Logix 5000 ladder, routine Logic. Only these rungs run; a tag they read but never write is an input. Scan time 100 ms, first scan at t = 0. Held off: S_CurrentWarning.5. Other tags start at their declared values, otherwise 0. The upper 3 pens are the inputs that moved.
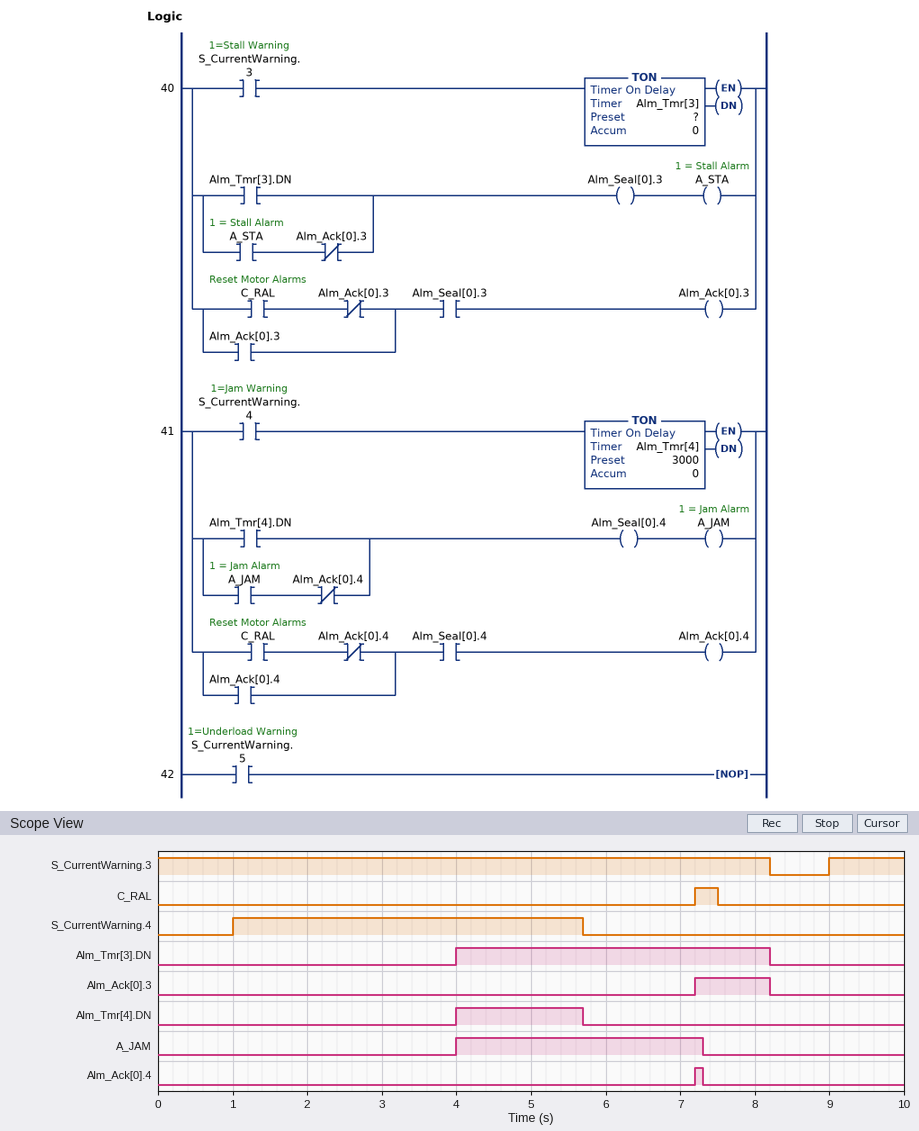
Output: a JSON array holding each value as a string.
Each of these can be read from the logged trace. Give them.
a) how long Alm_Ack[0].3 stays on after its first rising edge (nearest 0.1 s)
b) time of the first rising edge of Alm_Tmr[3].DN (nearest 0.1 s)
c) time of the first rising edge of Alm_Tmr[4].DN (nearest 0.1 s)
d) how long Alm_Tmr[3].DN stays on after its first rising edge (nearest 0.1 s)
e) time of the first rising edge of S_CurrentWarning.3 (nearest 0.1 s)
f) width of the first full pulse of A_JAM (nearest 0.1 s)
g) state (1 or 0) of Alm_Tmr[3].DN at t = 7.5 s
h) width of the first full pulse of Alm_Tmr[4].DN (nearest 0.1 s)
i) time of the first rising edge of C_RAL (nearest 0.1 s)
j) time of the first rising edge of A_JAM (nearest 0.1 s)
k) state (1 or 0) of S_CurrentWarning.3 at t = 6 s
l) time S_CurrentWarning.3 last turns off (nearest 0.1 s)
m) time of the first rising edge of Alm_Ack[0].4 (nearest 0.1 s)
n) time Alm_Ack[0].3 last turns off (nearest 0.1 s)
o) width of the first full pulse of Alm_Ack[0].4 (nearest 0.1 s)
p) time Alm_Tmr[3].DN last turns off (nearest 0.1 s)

["1.0 s", "4.0 s", "4.0 s", "4.2 s", "9.0 s", "3.3 s", "1", "1.7 s", "7.2 s", "4.0 s", "1", "8.2 s", "7.2 s", "8.2 s", "0.1 s", "8.2 s"]
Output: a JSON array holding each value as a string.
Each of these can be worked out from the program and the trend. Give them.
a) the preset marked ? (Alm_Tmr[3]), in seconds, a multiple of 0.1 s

["4.0 s"]
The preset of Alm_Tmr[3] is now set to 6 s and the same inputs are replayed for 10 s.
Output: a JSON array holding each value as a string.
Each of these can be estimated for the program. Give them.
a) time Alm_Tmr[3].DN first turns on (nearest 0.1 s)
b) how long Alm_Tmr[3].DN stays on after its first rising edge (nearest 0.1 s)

["6.0 s", "2.2 s"]
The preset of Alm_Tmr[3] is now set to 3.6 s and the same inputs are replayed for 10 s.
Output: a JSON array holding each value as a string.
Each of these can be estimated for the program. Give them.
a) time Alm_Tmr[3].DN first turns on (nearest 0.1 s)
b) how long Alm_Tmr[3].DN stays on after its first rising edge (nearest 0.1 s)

["3.6 s", "4.6 s"]
